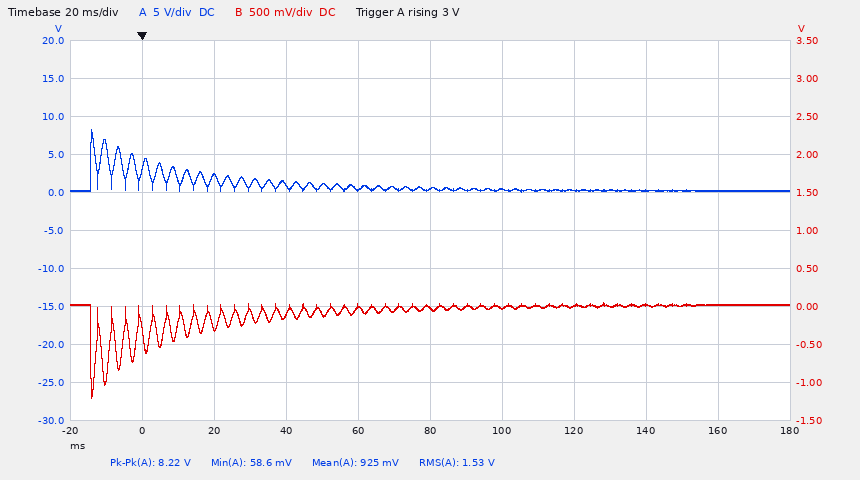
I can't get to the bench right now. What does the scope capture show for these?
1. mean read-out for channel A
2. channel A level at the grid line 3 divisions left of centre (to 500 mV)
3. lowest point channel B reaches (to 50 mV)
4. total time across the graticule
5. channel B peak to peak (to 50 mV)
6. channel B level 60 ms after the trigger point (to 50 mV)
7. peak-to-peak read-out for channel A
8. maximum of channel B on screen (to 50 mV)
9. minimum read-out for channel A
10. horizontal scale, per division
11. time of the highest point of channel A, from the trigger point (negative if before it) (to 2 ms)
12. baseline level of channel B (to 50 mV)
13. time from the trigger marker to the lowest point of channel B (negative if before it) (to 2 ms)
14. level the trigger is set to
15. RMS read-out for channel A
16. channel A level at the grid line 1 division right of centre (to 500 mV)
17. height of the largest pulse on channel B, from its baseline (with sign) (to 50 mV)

925 mV
2.0 V
-1.20 V
200 ms
1.25 V
0 mV
8.22 V
50 mV
58.6 mV
20 ms
-14 ms
0 mV
-14 ms
3 V
1.53 V
500 mV
-1.20 V
